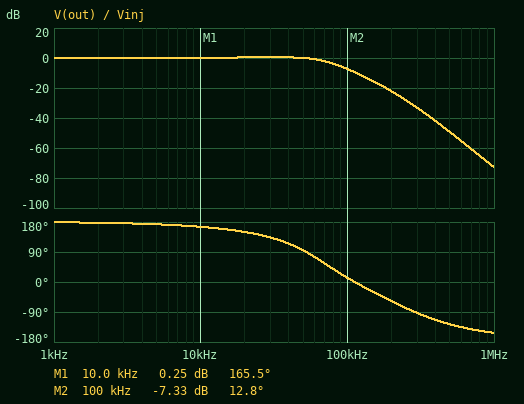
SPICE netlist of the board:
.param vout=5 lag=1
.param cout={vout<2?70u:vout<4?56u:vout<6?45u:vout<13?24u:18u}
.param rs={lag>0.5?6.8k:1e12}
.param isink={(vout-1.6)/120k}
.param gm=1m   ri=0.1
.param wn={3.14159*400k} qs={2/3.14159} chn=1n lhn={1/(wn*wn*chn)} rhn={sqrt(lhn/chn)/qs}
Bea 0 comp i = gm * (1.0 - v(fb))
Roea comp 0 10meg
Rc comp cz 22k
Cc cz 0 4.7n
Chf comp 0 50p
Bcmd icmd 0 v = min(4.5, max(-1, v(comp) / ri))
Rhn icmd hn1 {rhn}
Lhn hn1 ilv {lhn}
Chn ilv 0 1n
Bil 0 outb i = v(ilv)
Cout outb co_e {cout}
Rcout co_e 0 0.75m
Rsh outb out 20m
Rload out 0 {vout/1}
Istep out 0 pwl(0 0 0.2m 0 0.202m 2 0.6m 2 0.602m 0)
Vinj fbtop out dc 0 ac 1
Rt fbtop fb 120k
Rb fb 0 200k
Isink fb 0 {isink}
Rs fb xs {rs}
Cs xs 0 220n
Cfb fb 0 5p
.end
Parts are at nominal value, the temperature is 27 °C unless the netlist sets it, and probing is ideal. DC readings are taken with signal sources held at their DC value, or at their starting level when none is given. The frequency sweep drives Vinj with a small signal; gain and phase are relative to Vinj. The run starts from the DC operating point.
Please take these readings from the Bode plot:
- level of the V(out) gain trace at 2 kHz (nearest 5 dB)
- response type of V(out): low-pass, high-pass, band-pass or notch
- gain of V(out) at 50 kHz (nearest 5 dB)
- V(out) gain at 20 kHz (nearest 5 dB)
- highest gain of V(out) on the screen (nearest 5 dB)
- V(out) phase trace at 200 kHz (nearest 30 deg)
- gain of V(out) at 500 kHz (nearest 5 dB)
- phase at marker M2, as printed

0 dB
low-pass
0 dB
0 dB
0 dB
-60 deg
-50 dB
12.8 deg
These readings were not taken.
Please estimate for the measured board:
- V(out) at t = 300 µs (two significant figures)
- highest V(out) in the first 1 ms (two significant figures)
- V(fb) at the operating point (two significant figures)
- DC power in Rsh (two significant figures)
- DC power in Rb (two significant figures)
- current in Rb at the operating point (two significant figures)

4.9 V
5.2 V
1.0 V
20 mW
5.0 µW
5.0 µA
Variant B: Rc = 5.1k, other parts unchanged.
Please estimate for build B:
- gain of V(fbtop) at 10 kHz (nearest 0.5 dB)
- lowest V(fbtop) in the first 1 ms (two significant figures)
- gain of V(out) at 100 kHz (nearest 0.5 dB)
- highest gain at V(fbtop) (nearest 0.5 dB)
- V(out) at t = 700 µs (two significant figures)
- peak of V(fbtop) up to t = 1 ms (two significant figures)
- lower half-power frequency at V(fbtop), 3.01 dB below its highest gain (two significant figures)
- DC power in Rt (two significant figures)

0.5 dB
4.5 V
-21.0 dB
1.0 dB
5.0 V
5.5 V
7.4 kHz
130 µW
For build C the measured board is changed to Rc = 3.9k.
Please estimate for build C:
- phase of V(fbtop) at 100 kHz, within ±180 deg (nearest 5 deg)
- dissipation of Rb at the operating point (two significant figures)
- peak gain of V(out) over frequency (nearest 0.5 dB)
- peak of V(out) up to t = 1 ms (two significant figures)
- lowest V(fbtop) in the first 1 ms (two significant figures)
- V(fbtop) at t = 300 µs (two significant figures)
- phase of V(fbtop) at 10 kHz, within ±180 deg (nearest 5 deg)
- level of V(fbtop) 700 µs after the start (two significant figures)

0 deg
5.0 µW
3.5 dB
5.5 V
4.5 V
5.1 V
60 deg
4.9 V
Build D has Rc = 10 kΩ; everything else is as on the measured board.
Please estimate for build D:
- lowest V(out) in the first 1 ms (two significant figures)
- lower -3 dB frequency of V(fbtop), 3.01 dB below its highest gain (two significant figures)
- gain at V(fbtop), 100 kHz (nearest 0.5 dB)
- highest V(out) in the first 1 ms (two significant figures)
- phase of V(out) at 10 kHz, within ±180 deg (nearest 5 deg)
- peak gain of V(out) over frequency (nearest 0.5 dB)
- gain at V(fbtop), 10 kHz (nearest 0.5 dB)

4.7 V
17 kHz
1.5 dB
5.3 V
150 deg
1.0 dB
-5.0 dB
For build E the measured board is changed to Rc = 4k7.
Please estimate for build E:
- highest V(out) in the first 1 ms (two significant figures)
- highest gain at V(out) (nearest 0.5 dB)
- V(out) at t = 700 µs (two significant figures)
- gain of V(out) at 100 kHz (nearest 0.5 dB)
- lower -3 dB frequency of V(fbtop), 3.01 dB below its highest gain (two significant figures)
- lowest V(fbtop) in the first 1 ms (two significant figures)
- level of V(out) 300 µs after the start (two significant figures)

5.5 V
3.0 dB
4.9 V
-21.5 dB
7.2 kHz
4.5 V
5.1 V
